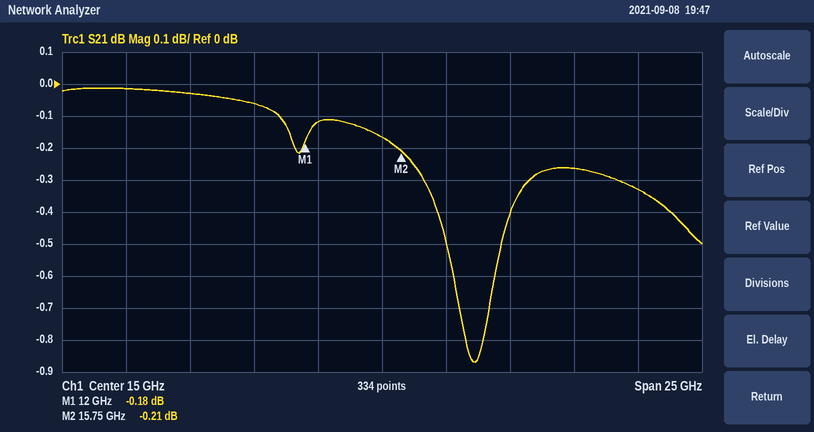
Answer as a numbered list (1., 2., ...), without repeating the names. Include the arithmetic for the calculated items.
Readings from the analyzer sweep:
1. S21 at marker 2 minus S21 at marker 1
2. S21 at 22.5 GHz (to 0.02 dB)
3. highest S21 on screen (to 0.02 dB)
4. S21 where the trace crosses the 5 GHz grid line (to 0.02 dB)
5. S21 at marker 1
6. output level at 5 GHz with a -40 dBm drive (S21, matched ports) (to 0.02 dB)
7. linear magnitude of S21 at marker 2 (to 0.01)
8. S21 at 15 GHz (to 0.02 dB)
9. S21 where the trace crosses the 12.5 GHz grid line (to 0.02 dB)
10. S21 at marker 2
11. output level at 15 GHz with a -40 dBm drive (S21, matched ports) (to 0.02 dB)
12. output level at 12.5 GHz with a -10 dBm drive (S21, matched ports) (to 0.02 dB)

1. -0.21 − (-0.18) = -0.03 dB
2. -0.26 dB
3. -0.02 dB
4. -0.02 dB
5. -0.18 dB
6. -40 dBm + (-0.02 dB) = -40.02 dBm
7. 10^(-0.21/20) ≈ 0.98
8. -0.16 dB
9. -0.12 dB
10. -0.21 dB
11. -40 dBm + (-0.16 dB) = -40.16 dBm
12. -10 dBm + (-0.12 dB) = -10.12 dBm
